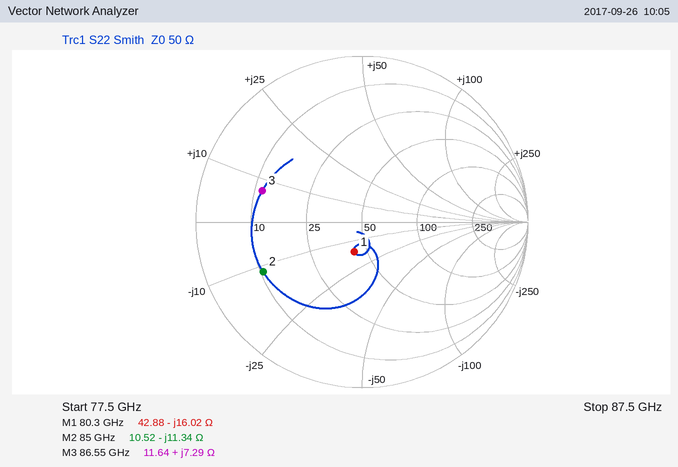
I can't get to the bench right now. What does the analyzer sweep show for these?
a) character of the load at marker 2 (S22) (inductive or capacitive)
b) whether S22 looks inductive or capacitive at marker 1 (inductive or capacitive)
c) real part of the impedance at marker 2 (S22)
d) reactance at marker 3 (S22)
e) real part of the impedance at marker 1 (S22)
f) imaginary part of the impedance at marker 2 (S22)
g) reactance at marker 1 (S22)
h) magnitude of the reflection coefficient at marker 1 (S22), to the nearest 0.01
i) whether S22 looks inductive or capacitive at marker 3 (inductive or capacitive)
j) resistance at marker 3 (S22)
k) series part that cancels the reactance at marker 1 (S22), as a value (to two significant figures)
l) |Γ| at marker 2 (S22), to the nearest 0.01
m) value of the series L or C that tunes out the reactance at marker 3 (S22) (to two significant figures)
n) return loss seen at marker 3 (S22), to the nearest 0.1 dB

capacitive
capacitive
10.52 Ω
+7.29 Ω
42.88 Ω
-11.34 Ω
-16.02 Ω
0.19
inductive
11.64 Ω
32 pH
0.67
250 fF
4.0 dB
